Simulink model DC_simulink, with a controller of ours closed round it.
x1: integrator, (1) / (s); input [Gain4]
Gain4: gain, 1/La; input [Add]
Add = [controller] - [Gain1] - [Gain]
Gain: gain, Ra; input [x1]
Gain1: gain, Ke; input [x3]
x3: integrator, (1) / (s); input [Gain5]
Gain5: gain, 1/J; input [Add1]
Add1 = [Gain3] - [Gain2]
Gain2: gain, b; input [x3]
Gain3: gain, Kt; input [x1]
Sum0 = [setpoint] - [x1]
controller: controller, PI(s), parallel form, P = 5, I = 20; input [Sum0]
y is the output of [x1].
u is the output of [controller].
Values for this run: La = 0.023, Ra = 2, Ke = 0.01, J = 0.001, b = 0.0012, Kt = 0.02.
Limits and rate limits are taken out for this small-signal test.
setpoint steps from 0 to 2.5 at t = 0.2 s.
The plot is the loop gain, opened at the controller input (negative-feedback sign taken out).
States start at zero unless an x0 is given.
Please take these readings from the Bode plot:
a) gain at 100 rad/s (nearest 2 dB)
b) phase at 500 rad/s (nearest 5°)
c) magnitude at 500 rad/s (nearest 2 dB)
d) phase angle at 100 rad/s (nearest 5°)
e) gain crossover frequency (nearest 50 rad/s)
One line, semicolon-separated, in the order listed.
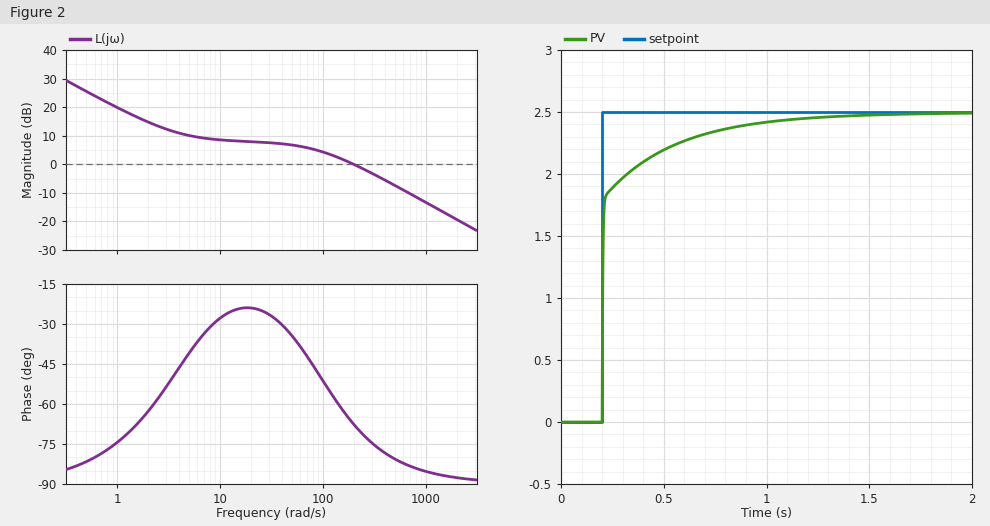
4 dB; -80°; -8 dB; -50°; 200 rad/s
